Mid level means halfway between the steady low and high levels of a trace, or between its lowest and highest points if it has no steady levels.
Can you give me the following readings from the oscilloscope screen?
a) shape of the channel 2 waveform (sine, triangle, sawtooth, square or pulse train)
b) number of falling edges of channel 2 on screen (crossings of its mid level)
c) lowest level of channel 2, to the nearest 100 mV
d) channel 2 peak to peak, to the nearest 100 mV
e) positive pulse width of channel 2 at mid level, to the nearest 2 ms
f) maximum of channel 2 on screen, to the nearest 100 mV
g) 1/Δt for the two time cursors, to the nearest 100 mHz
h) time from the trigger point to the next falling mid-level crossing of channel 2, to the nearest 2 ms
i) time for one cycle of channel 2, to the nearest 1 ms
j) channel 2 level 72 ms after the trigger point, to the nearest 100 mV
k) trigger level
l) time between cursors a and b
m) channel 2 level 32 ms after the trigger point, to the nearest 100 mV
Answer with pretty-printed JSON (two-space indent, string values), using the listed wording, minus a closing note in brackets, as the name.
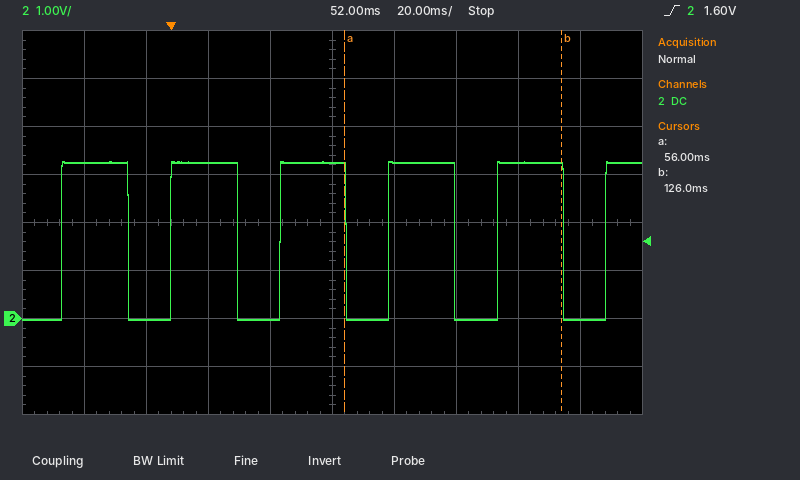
{
  "shape of the channel 2 waveform": "pulse train",
  "number of falling edges of channel 2 on screen": "5",
  "lowest level of channel 2, to the nearest 100 mV": "0.0 V",
  "channel 2 peak to peak, to the nearest 100 mV": "3.3 V",
  "positive pulse width of channel 2 at mid level, to the nearest 2 ms": "22 ms",
  "maximum of channel 2 on screen, to the nearest 100 mV": "3.3 V",
  "1/Δt for the two time cursors, to the nearest 100 mHz": "14.3 Hz",
  "time from the trigger point to the next falling mid-level crossing of channel 2, to the nearest 2 ms": "22 ms",
  "time for one cycle of channel 2, to the nearest 1 ms": "35 ms",
  "channel 2 level 72 ms after the trigger point, to the nearest 100 mV": "3.3 V",
  "trigger level": "1.60 V",
  "time between cursors a and b": "70 ms",
  "channel 2 level 32 ms after the trigger point, to the nearest 100 mV": "0.0 V"
}
